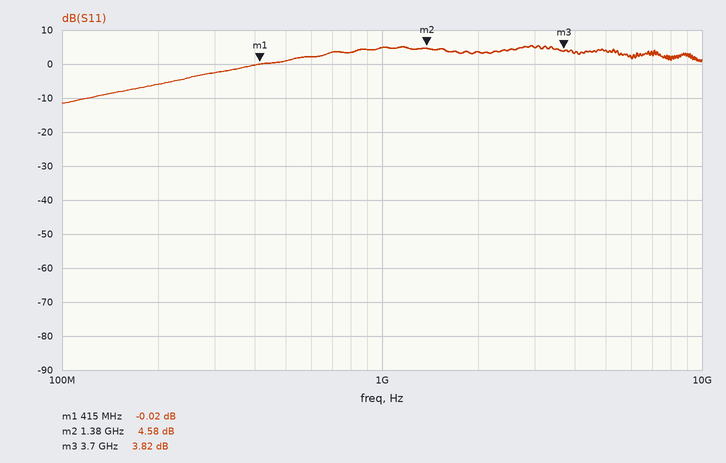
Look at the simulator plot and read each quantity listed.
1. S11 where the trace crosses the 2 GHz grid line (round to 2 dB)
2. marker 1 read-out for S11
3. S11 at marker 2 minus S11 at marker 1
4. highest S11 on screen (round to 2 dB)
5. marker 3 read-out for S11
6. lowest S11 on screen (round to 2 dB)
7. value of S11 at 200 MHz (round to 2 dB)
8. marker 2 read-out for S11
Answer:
4 dB
-0.02 dB
4.60 dB
6 dB
3.82 dB
-12 dB
-6 dB
4.58 dB
